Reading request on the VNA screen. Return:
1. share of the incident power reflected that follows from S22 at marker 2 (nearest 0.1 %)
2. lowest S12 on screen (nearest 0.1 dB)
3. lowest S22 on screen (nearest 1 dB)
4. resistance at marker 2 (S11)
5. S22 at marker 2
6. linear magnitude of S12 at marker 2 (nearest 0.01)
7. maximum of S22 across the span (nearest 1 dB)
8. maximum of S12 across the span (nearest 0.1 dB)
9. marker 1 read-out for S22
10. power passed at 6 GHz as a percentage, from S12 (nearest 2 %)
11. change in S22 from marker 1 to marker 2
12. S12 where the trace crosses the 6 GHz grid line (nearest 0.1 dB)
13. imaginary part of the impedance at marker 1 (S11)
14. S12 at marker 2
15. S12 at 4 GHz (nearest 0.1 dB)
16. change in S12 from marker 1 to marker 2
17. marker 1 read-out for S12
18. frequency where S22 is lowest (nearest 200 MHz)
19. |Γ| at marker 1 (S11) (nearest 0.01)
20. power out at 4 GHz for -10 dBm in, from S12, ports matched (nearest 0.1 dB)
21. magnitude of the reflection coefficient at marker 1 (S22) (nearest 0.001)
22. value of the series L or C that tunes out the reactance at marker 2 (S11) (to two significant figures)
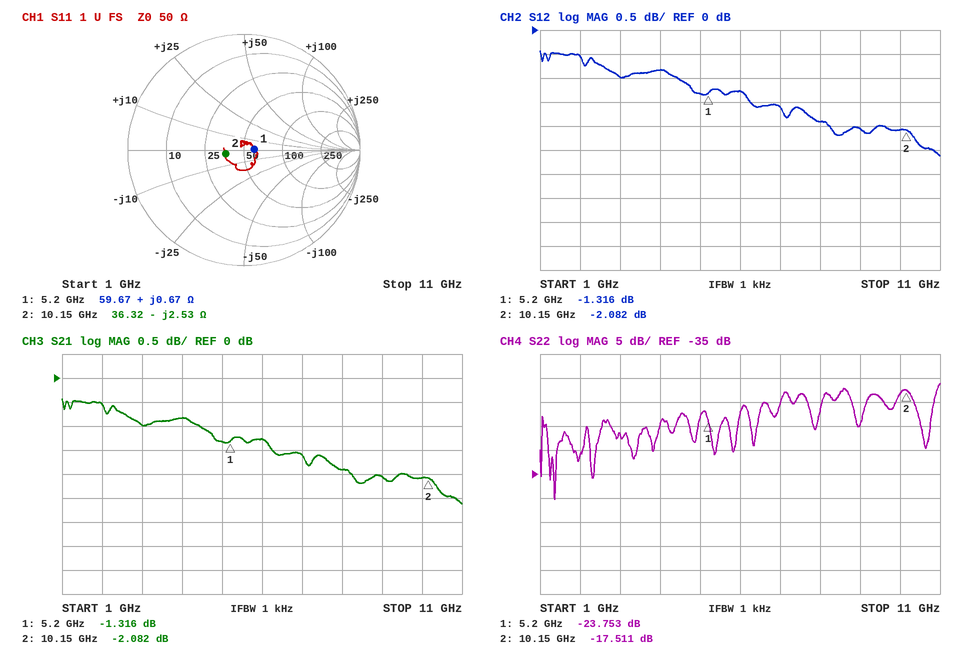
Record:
1.8 %
-2.6 dB
-40 dB
36.32 Ω
-17.511 dB
0.79
-16 dB
-0.4 dB
-23.753 dB
74 %
6.242 dB
-1.3 dB
+0.67 Ω
-2.082 dB
-0.8 dB
-0.766 dB
-1.316 dB
1.4 GHz
0.09
-10.8 dBm
0.065
40 pH
